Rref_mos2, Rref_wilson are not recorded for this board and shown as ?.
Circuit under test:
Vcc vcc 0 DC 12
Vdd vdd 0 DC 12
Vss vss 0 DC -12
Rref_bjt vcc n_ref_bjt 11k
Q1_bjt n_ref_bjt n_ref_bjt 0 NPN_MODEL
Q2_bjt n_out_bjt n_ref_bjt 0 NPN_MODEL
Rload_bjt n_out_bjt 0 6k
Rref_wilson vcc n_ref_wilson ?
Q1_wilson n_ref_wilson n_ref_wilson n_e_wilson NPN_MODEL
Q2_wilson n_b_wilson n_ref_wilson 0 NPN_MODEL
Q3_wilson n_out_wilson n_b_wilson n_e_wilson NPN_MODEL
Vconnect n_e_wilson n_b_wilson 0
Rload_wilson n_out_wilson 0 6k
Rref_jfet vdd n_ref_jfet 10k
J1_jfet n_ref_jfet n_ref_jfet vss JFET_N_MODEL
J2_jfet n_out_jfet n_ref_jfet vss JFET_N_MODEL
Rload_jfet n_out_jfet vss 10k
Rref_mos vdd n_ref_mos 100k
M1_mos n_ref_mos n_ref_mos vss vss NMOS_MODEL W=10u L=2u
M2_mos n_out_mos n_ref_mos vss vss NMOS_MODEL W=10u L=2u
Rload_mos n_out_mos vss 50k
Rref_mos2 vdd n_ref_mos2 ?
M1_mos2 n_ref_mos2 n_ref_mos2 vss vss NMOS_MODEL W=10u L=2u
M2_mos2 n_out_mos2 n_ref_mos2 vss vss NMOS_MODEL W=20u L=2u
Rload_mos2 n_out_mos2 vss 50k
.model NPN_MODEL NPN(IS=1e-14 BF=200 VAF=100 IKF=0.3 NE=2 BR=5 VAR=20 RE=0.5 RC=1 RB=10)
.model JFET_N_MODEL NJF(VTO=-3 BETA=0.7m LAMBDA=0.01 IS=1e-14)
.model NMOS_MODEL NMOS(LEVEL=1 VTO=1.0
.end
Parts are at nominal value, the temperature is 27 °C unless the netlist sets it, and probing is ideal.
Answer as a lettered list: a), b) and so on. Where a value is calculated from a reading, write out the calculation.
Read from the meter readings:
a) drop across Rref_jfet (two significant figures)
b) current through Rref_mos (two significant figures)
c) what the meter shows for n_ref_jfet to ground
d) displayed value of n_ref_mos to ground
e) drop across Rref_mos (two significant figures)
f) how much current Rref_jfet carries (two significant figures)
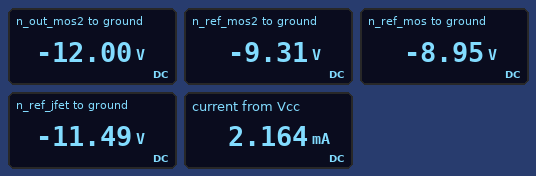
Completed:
a) 12 V - (-11.49 V) = 23 V
b) (12 V - (-8.95 V)) / 100 kΩ = 210 µA
c) -11.49 V
d) -8.95 V
e) 12 V - (-8.95 V) = 21 V
f) (12 V - (-11.49 V)) / 10 kΩ = 2.3 mA
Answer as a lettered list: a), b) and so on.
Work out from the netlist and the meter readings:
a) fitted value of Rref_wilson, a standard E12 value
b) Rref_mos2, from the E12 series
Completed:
a) 10 kΩ
b) 150 kΩ
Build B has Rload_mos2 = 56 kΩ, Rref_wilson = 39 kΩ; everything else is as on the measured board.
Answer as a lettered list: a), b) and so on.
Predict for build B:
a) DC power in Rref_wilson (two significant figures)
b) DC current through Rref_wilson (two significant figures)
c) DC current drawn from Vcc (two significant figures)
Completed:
a) 3.3 mW
b) 290 µA
c) 1.3 mA
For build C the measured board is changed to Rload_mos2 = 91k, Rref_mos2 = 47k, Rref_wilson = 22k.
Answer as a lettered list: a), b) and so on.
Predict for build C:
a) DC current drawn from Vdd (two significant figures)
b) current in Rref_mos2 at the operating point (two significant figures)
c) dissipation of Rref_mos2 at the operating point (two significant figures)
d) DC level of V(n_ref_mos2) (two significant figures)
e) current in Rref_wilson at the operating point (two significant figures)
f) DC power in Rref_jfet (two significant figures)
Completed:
a) 3.0 mA
b) 430 µA
c) 8.6 mW
d) -8.1 V
e) 520 µA
f) 55 mW
